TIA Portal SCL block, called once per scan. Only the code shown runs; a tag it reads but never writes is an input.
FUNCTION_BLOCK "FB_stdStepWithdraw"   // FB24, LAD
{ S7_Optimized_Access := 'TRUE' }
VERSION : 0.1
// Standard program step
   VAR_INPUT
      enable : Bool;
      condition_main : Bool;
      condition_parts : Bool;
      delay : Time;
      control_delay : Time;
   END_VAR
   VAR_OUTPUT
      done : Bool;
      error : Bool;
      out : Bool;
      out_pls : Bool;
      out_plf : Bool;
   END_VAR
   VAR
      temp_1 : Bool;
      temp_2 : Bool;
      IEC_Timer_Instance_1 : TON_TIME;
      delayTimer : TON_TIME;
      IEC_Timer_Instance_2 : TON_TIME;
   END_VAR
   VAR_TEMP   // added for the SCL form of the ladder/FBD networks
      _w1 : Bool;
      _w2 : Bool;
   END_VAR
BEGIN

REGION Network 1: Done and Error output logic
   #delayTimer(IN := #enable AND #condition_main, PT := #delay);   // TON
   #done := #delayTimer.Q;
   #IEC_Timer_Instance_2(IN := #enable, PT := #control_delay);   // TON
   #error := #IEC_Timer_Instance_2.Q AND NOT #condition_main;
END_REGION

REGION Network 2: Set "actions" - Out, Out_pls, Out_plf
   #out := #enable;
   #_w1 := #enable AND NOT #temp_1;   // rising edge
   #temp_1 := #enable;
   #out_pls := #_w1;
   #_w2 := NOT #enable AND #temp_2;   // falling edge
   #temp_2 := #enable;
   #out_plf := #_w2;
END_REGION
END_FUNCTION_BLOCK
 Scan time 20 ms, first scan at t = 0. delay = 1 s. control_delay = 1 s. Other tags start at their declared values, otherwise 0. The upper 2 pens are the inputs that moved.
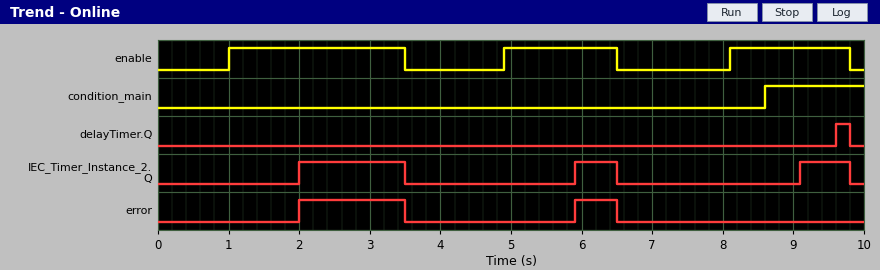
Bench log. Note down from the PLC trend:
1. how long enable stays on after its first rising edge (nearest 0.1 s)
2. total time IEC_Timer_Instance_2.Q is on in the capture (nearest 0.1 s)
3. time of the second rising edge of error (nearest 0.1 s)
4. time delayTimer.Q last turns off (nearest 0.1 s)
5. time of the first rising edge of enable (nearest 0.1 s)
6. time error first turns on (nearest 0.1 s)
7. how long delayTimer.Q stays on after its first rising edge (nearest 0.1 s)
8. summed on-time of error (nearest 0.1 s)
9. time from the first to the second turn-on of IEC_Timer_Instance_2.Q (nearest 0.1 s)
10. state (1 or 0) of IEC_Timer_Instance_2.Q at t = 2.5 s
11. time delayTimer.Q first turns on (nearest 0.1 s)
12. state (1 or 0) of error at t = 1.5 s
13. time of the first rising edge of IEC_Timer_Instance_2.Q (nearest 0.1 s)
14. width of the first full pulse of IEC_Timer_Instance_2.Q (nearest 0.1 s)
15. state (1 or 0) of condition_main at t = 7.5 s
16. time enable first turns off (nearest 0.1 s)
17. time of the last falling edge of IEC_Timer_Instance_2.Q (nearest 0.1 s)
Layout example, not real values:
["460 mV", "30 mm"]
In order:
["2.5 s", "2.8 s", "5.9 s", "9.8 s", "1.0 s", "2.0 s", "0.2 s", "2.1 s", "3.9 s", "1", "9.6 s", "0", "2.0 s", "1.5 s", "0", "3.5 s", "9.8 s"]
